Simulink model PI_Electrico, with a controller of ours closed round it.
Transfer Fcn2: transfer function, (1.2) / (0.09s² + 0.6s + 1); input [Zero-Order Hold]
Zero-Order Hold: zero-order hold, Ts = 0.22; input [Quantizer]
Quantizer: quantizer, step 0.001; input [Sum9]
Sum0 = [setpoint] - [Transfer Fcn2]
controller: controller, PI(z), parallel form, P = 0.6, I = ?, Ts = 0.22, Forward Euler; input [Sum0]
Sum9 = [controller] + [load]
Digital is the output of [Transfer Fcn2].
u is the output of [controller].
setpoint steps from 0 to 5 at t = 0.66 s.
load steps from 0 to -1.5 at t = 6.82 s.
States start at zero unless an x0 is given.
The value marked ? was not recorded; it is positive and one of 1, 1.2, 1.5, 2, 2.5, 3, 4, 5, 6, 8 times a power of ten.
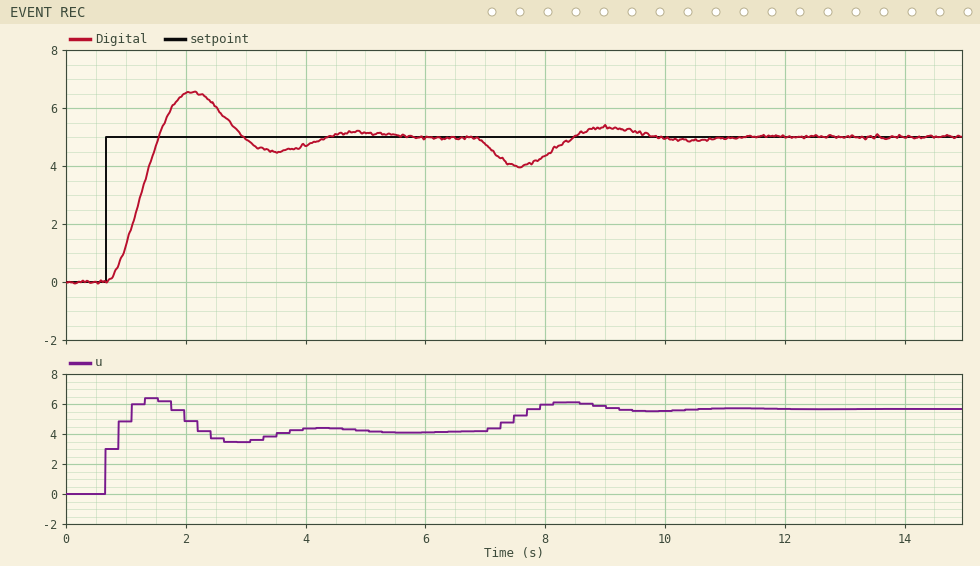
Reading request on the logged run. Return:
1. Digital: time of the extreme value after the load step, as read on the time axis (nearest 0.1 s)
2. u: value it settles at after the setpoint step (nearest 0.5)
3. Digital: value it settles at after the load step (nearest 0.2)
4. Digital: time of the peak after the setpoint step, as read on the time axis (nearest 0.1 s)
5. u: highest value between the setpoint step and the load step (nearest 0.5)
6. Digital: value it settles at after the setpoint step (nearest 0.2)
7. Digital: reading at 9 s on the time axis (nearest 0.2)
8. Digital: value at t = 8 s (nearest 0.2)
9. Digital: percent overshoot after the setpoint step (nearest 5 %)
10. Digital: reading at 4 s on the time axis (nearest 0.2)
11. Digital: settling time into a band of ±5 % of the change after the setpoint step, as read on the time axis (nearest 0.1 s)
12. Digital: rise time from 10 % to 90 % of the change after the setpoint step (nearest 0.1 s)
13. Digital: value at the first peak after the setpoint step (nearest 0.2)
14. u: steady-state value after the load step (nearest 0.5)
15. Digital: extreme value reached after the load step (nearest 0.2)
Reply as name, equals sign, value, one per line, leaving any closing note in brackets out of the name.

Digital: time of the extreme value after the load step, as read on the time axis = 7.6 s
u: value it settles at after the setpoint step = 4.0
Digital: value it settles at after the load step = 5.0
Digital: time of the peak after the setpoint step, as read on the time axis = 2.1 s
u: highest value between the setpoint step and the load step = 6.5
Digital: value it settles at after the setpoint step = 5.0
Digital: reading at 9 s on the time axis = 5.4
Digital: value at t = 8 s = 4.4
Digital: percent overshoot after the setpoint step = 30 %
Digital: reading at 4 s on the time axis = 4.8
Digital: settling time into a band of ±5 % of the change after the setpoint step, as read on the time axis = 4.0 s
Digital: rise time from 10 % to 90 % of the change after the setpoint step = 0.6 s
Digital: value at the first peak after the setpoint step = 6.6
u: steady-state value after the load step = 5.5
Digital: extreme value reached after the load step = 4.0
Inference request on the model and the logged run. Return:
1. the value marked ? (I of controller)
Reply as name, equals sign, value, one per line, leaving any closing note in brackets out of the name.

the value marked ? = 2
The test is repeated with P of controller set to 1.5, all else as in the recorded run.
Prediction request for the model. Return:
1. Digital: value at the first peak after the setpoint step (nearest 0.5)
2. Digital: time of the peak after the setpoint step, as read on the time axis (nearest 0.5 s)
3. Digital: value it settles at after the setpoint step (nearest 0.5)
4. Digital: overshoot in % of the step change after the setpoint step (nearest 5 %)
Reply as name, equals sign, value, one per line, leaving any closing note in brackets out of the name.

Digital: value at the first peak after the setpoint step = 5.5
Digital: time of the peak after the setpoint step, as read on the time axis = 1.5 s
Digital: value it settles at after the setpoint step = 5.0
Digital: overshoot in % of the step change after the setpoint step = 15 %
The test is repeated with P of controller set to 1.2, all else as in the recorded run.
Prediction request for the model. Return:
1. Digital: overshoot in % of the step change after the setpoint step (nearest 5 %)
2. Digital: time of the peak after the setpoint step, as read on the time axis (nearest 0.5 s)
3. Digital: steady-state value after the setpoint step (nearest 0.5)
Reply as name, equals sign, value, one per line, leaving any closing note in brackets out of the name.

Digital: overshoot in % of the step change after the setpoint step = 15 %
Digital: time of the peak after the setpoint step, as read on the time axis = 1.5 s
Digital: steady-state value after the setpoint step = 5.0
